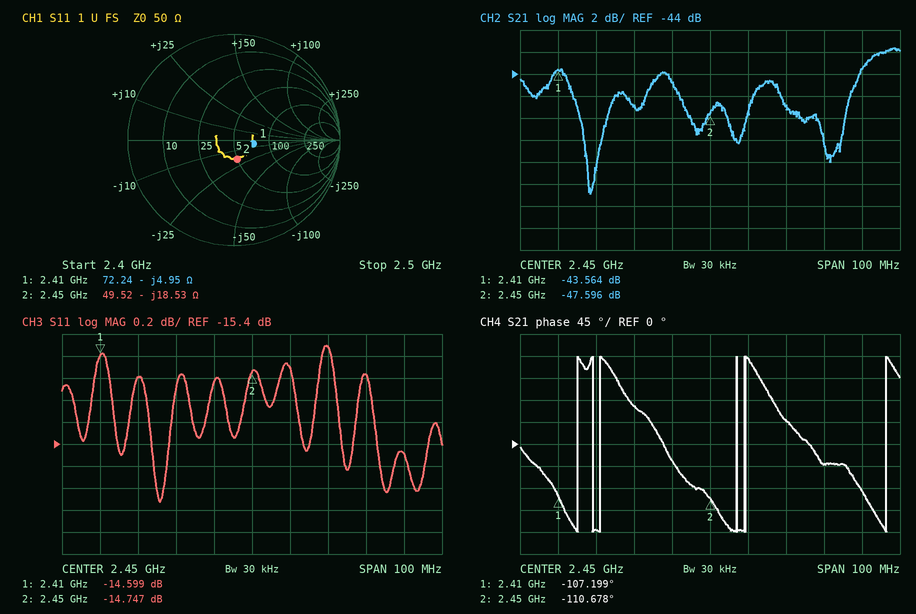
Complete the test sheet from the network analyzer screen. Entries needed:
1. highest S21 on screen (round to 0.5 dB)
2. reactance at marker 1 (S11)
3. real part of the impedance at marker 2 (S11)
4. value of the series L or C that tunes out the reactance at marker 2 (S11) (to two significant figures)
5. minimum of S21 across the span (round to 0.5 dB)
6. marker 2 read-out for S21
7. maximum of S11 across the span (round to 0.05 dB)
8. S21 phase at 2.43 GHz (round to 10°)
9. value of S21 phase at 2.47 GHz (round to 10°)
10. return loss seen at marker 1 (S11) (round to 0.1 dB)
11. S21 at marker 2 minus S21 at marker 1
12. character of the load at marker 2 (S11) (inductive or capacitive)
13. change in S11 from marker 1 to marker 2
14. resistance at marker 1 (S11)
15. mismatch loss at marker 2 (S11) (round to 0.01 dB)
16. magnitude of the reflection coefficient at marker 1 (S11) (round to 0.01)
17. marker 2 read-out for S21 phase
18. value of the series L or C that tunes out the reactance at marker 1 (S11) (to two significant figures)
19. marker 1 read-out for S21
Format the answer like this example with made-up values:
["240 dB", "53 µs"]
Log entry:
["-41.5 dB", "-4.95 Ω", "49.52 Ω", "1.2 nH", "-55.0 dB", "-47.596 dB", "-14.50 dB", "80°", "50°", "14.6 dB", "-4.032 dB", "capacitive", "-0.148 dB", "72.24 Ω", "0.15 dB", "0.19", "-110.678°", "330 pH", "-43.564 dB"]
